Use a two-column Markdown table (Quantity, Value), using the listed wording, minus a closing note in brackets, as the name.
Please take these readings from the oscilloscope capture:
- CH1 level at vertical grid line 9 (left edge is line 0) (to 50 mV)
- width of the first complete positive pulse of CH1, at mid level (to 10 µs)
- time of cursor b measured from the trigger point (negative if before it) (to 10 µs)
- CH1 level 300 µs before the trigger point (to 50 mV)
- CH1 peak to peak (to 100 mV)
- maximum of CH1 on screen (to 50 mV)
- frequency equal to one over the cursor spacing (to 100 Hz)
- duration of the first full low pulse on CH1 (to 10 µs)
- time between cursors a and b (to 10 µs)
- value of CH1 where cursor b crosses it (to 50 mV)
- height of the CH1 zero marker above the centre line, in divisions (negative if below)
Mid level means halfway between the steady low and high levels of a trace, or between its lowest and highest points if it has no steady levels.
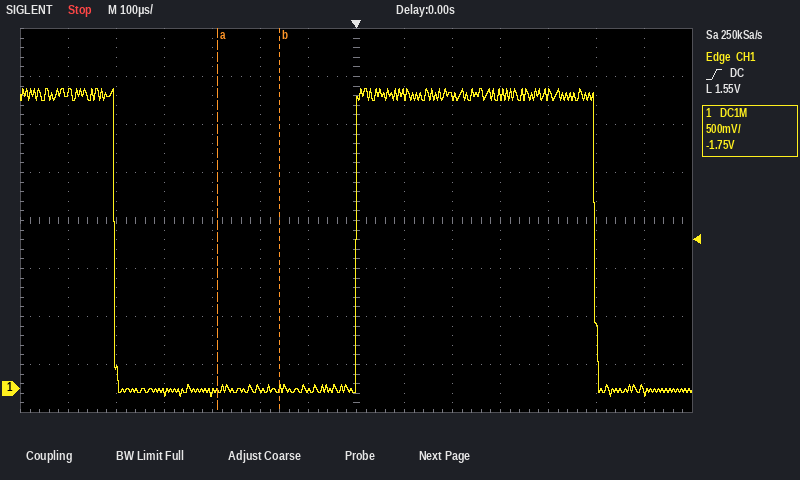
| Quantity | Value |
|---|---|
| CH1 level at vertical grid line 9 (left edge is line 0) | 3.05 V |
| width of the first complete positive pulse of CH1, at mid level | 500 µs |
| time of cursor b measured from the trigger point (negative if before it) | -160 µs |
| CH1 level 300 µs before the trigger point | -50 mV |
| CH1 peak to peak | 3.20 V |
| maximum of CH1 on screen | 3.10 V |
| frequency equal to one over the cursor spacing | 7.7 kHz |
| duration of the first full low pulse on CH1 | 500 µs |
| time between cursors a and b | 130 µs |
| value of CH1 where cursor b crosses it | 0 mV |
| height of the CH1 zero marker above the centre line, in divisions | -3.5 div |
